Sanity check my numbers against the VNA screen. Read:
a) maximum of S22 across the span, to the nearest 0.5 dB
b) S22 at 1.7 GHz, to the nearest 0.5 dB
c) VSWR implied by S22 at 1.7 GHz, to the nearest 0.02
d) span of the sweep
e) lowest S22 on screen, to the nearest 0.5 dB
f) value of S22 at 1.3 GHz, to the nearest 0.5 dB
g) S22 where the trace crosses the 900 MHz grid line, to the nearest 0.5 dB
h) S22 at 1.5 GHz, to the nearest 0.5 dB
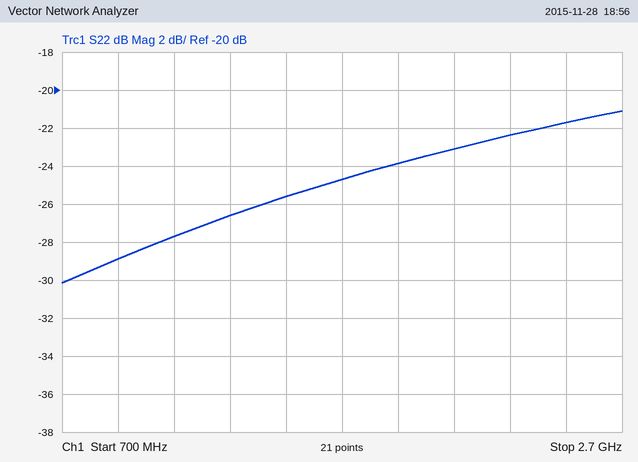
-21.0 dB
-24.5 dB
1.12
2 GHz
-30.0 dB
-26.5 dB
-29.0 dB
-25.5 dB
